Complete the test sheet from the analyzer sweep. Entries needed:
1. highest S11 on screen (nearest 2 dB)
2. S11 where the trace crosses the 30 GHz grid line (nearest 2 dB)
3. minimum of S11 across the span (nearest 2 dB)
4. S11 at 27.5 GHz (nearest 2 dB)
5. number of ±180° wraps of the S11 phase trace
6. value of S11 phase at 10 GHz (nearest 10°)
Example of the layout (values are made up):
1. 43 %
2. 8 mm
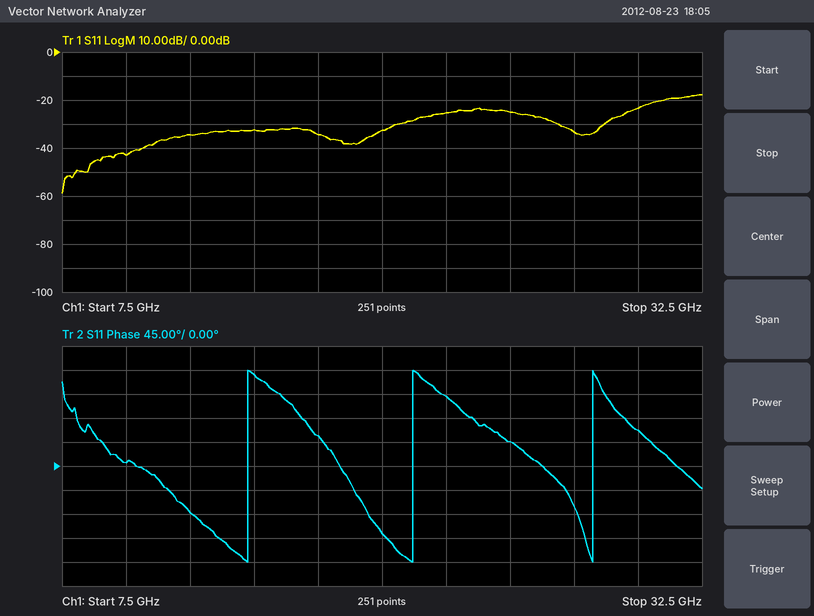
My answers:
1. -18 dB
2. -24 dB
3. -58 dB
4. -34 dB
5. 3
6. 10°
